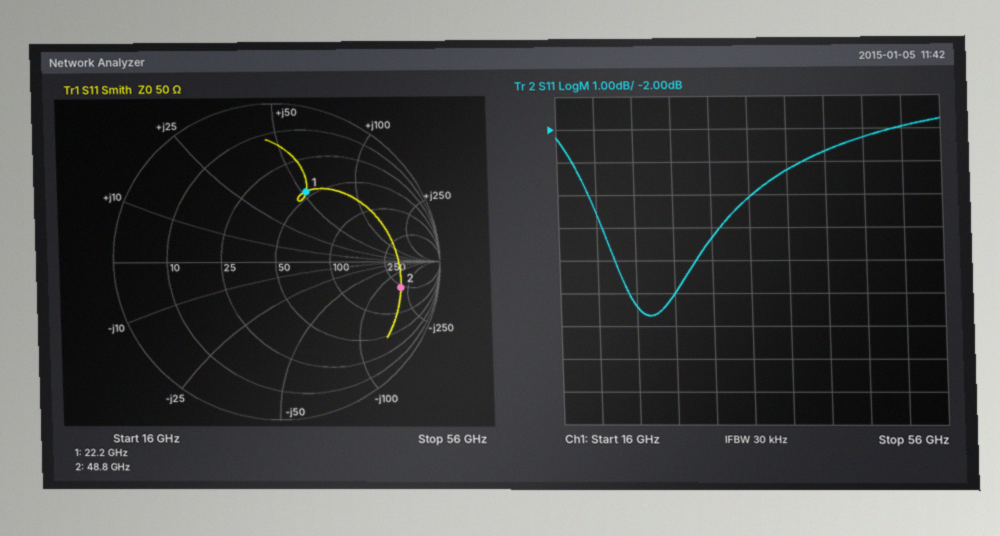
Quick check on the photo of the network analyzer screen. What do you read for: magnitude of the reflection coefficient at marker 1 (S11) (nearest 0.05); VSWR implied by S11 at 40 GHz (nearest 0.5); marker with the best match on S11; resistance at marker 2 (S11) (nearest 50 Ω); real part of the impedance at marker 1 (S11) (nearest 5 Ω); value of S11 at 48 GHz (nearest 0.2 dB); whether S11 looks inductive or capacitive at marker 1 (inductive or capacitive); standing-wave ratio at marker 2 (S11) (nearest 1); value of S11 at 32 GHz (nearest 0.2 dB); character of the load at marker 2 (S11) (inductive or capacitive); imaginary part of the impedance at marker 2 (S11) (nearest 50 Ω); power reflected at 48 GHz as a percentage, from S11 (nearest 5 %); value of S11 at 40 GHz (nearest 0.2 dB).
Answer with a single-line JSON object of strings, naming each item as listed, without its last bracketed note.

{"magnitude of the reflection coefficient at marker 1 (S11)": "0.50", "VSWR implied by S11 at 40 GHz": "5.5", "marker with the best match on S11": "marker 1", "resistance at marker 2 (S11)": "250 Ω", "real part of the impedance at marker 1 (S11)": "45 Ω", "value of S11 at 48 GHz": "-2.2 dB", "whether S11 looks inductive or capacitive at marker 1": "inductive", "standing-wave ratio at marker 2 (S11)": "8", "value of S11 at 32 GHz": "-5.4 dB", "character of the load at marker 2 (S11)": "capacitive", "imaginary part of the impedance at marker 2 (S11)": "-200 Ω", "power reflected at 48 GHz as a percentage, from S11": "60 %", "value of S11 at 40 GHz": "-3.2 dB"}
